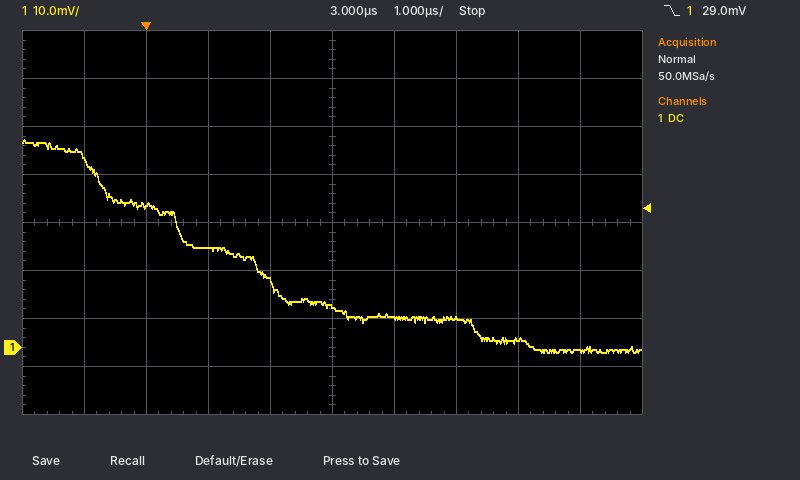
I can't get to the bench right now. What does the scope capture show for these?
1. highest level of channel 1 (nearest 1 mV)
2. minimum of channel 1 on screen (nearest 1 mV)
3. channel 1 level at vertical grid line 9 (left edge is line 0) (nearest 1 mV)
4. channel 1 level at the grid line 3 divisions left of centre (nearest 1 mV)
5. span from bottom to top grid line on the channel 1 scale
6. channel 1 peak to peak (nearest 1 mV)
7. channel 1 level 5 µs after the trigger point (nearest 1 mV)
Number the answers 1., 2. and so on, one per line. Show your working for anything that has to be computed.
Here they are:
1. 43 mV
2. -1 mV
3. -1 mV
4. 30 mV
5. 80 mV
6. 43 mV − (-1 mV) = 44 mV
7. 6 mV
